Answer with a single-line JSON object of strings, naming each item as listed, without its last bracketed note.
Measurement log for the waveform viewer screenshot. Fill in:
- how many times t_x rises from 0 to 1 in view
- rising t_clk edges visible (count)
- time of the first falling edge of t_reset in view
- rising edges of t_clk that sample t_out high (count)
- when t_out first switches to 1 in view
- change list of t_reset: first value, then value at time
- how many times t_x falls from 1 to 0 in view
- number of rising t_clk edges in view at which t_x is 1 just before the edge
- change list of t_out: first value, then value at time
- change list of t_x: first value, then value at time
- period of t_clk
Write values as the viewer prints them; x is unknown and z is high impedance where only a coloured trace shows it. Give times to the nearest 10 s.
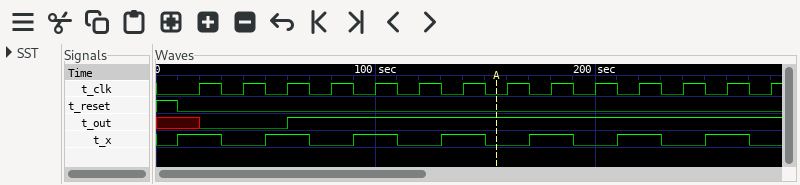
{"how many times t_x rises from 0 to 1 in view": "7", "rising t_clk edges visible": "14", "time of the first falling edge of t_reset in view": "10 s", "rising edges of t_clk that sample t_out high": "11", "when t_out first switches to 1 in view": "60 s", "change list of t_reset: first value, then value at time": "1, 0 at 10 s", "how many times t_x falls from 1 to 0 in view": "7", "number of rising t_clk edges in view at which t_x is 1 just before the edge": "7", "change list of t_out: first value, then value at time": "x, 0 at 20 s, 1 at 60 s", "change list of t_x: first value, then value at time": "0, 1 at 10 s, 0 at 30 s, 1 at 50 s, 0 at 70 s, 1 at 90 s, 0 at 110 s, 1 at 130 s, 0 at 150 s, 1 at 170 s, 0 at 190 s, 1 at 210 s, 0 at 230 s, 1 at 250 s, 0 at 270 s", "period of t_clk": "20 s"}
